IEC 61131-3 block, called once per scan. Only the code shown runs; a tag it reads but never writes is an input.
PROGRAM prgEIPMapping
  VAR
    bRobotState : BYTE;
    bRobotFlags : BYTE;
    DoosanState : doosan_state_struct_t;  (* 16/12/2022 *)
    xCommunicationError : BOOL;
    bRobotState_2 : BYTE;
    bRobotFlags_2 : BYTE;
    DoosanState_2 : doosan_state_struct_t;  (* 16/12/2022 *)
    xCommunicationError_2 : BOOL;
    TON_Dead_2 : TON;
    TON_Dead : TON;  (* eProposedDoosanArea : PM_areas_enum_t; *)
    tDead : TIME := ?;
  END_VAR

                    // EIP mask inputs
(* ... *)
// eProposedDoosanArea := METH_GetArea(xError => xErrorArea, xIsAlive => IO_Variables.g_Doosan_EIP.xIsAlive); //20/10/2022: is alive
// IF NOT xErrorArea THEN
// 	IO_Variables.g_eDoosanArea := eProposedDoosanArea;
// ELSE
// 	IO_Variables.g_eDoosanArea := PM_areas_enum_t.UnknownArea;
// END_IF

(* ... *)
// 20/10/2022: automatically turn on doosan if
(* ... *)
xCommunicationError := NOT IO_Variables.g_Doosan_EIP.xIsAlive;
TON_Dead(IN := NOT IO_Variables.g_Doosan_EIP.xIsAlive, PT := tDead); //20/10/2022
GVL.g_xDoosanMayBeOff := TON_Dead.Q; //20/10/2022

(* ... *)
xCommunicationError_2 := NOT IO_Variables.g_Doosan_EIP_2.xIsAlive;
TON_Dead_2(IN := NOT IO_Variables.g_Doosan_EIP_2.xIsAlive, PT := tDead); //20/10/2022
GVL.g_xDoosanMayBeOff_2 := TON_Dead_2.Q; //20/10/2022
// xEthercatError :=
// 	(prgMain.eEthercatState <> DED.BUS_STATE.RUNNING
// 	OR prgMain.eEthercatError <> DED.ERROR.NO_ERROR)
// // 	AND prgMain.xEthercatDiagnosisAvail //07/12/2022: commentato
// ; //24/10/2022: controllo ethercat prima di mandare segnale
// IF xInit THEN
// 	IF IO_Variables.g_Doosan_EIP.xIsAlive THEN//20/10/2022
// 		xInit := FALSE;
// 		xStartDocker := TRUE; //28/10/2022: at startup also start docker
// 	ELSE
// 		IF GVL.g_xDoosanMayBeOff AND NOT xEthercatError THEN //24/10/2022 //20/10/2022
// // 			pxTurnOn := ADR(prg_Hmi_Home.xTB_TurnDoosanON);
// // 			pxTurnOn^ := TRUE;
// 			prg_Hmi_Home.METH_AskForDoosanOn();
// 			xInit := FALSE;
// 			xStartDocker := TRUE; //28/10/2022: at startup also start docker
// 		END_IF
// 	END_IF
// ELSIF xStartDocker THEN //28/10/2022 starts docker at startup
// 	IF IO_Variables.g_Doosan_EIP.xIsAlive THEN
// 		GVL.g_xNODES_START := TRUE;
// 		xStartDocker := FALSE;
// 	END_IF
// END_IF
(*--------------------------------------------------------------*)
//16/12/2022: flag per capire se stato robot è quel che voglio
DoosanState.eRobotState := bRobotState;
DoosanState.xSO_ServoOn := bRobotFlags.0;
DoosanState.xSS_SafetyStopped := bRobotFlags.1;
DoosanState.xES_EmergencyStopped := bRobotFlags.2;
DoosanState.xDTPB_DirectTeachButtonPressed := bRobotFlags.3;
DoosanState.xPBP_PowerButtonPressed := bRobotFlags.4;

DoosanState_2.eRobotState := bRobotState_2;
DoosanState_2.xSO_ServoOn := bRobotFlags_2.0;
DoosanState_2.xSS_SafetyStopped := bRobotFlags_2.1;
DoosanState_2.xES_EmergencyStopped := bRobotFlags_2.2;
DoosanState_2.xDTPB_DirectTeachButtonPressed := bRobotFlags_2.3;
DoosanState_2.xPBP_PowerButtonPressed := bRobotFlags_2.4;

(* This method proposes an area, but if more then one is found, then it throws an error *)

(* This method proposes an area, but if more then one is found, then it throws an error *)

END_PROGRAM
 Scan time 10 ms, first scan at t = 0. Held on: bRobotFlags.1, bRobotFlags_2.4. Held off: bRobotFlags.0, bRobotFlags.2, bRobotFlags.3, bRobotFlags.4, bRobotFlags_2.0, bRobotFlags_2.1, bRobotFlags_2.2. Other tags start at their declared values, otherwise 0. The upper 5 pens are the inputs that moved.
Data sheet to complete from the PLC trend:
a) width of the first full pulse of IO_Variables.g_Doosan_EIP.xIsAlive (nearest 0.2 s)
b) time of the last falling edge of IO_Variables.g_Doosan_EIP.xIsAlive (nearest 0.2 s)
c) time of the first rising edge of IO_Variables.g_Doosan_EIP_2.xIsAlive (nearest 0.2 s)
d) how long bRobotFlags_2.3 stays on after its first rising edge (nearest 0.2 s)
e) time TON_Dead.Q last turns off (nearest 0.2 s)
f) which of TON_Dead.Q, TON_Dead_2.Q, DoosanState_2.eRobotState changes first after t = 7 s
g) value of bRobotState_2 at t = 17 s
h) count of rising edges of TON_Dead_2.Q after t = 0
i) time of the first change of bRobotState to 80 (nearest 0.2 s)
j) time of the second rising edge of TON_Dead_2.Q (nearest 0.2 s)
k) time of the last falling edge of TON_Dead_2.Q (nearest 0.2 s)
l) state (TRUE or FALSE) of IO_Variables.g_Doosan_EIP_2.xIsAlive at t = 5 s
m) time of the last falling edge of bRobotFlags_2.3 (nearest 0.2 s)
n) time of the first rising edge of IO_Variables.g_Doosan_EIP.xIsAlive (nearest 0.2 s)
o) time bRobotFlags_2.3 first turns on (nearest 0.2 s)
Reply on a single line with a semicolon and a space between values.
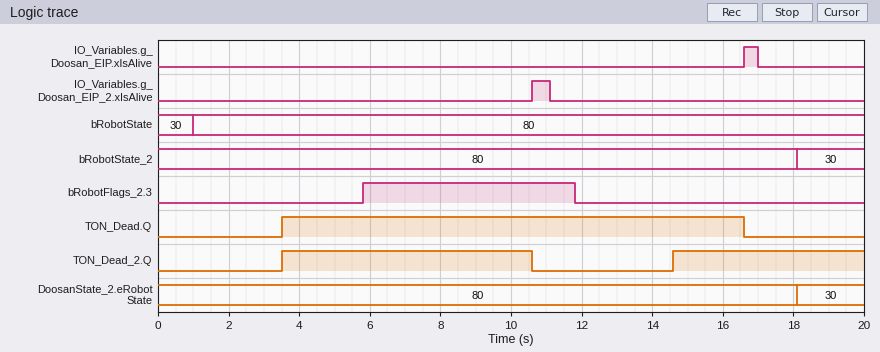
0.4 s; 17.0 s; 10.6 s; 6.0 s; 16.6 s; TON_Dead_2.Q; 80; 2; 1.0 s; 14.6 s; 10.6 s; FALSE; 11.8 s; 16.6 s; 5.8 s
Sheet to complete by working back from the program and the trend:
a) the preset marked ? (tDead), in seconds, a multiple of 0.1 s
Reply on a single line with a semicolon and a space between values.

3.5 s
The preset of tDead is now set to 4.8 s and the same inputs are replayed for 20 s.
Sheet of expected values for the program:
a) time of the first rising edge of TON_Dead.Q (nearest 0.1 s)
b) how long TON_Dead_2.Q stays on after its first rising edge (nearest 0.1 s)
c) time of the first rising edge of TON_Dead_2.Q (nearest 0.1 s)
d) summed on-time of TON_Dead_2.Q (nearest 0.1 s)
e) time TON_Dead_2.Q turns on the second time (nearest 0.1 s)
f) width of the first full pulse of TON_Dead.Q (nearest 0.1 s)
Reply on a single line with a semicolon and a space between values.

4.8 s; 5.8 s; 4.8 s; 9.9 s; 15.9 s; 11.8 s
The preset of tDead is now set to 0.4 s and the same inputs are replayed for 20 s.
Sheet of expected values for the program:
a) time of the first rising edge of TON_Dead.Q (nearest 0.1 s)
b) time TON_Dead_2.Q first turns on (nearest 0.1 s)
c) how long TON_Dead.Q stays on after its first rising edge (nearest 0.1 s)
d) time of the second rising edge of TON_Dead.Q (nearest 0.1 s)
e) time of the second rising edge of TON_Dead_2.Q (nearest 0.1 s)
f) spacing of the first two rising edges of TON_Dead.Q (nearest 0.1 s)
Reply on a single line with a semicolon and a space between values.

0.4 s; 0.4 s; 16.2 s; 17.4 s; 11.5 s; 17.0 s
